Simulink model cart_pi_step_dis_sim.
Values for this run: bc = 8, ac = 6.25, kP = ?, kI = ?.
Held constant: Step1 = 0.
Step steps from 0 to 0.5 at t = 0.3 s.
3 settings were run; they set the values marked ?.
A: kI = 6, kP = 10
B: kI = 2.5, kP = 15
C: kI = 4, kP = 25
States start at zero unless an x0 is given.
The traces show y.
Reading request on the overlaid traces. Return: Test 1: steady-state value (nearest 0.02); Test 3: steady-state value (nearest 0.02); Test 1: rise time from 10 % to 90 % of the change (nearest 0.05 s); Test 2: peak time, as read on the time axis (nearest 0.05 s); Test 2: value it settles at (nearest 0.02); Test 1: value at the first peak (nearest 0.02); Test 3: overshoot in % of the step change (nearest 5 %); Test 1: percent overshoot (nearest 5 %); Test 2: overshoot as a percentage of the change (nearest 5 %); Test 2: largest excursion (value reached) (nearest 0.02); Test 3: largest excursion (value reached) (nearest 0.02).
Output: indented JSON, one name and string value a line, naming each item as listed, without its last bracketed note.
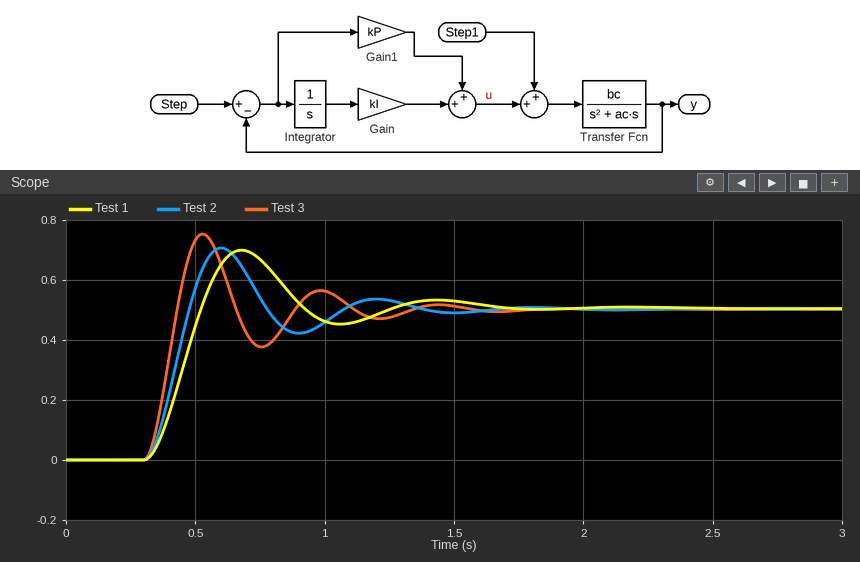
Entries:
{
  "Test 1: steady-state value": "0.50",
  "Test 3: steady-state value": "0.50",
  "Test 1: rise time from 10 % to 90 % of the change": "0.15 s",
  "Test 2: peak time, as read on the time axis": "0.60 s",
  "Test 2: value it settles at": "0.50",
  "Test 1: value at the first peak": "0.70",
  "Test 3: overshoot in % of the step change": "50 %",
  "Test 1: percent overshoot": "40 %",
  "Test 2: overshoot as a percentage of the change": "40 %",
  "Test 2: largest excursion (value reached)": "0.70",
  "Test 3: largest excursion (value reached)": "0.76"
}
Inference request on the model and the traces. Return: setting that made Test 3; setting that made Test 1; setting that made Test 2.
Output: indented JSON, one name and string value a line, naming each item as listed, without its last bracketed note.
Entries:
{
  "setting that made Test 3": "C",
  "setting that made Test 1": "A",
  "setting that made Test 2": "B"
}
